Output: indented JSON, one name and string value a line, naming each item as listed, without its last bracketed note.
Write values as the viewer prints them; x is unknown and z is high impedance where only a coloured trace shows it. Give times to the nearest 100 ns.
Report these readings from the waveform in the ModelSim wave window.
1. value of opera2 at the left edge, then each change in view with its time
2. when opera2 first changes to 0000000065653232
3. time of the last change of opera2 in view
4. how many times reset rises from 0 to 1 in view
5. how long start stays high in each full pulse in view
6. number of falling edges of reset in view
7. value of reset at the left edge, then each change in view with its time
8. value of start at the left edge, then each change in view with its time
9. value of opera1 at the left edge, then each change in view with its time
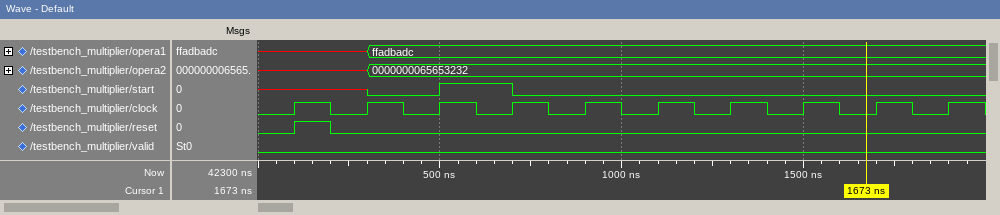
{
  "value of opera2 at the left edge, then each change in view with its time": "x, 0000000065653232 at 300 ns",
  "when opera2 first changes to 0000000065653232": "300 ns",
  "time of the last change of opera2 in view": "300 ns",
  "how many times reset rises from 0 to 1 in view": "1",
  "how long start stays high in each full pulse in view": "200 ns",
  "number of falling edges of reset in view": "1",
  "value of reset at the left edge, then each change in view with its time": "0, 1 at 100 ns, 0 at 200 ns",
  "value of start at the left edge, then each change in view with its time": "x, 0 at 300 ns, 1 at 500 ns, 0 at 700 ns",
  "value of opera1 at the left edge, then each change in view with its time": "x, ffadbadc at 300 ns"
}
